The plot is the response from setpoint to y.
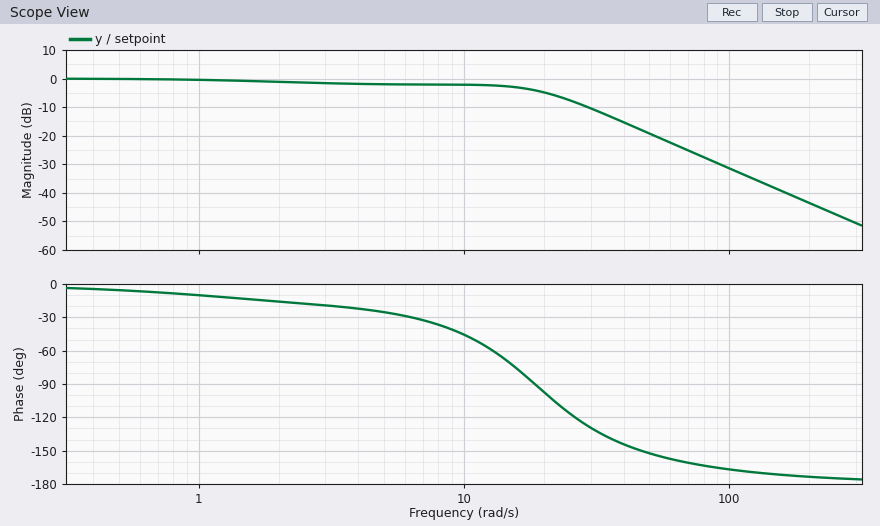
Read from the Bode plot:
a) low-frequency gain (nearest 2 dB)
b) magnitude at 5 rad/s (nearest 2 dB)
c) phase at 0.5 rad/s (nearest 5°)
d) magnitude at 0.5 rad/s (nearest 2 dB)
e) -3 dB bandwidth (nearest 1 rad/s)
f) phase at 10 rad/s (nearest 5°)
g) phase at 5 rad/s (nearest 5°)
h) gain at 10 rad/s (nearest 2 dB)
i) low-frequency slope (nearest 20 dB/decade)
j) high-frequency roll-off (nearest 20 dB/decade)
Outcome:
0 dB
-2 dB
-5°
0 dB
16 rad/s
-45°
-25°
-2 dB
0 dB/decade
-40 dB/decade
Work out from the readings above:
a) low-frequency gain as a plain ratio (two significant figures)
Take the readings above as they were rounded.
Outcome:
1.0
